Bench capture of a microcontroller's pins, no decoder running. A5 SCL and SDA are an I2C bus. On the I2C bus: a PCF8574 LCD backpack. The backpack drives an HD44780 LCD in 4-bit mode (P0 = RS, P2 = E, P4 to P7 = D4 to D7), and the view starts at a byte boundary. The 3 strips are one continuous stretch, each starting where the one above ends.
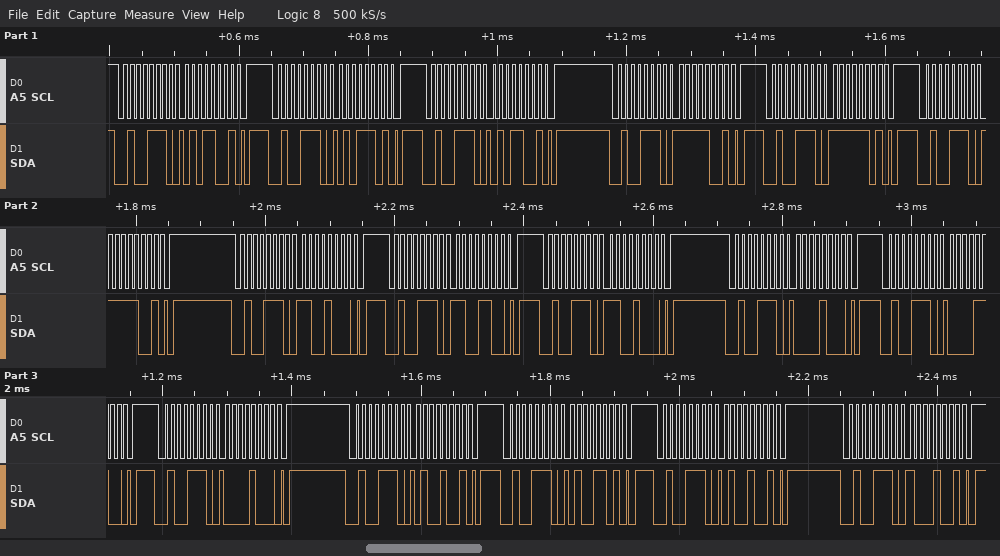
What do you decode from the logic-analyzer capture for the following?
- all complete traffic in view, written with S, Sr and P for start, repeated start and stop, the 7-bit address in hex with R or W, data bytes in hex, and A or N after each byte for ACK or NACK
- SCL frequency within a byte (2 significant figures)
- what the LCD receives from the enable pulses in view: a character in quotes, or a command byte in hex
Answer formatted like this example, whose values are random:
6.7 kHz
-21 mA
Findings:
S 27W A 59 A P S 27W A 5D A P S 27W A 59 A P S 27W A F9 A P S 27W A FD A P S 27W A F9 A P S 27W A C8 A P S 27W A CC A P S 27W A C8 A P S 27W A 08 A P S 27W A 0C A P S 27W A 08 A P S 27W A 49 A P S 27W A 4D A P S 27W A 49 A P S 27W A 89 A P
100 kHz
'_' 0xC0
